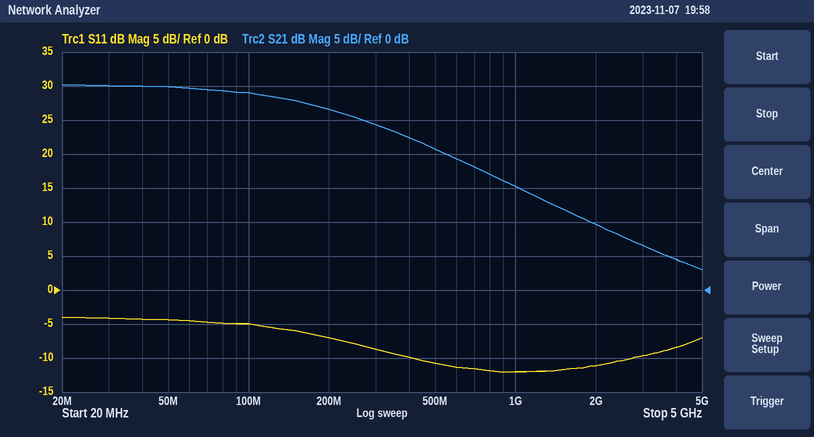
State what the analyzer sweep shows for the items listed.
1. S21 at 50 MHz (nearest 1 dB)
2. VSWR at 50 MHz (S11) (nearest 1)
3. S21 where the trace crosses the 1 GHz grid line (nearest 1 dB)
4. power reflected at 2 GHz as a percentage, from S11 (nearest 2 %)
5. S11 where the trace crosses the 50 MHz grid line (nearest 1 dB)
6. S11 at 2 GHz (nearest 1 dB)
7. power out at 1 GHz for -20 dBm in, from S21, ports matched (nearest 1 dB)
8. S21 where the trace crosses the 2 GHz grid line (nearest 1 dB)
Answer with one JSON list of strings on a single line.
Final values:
["30 dB", "4", "15 dB", "8 %", "-4 dB", "-11 dB", "-5 dBm", "10 dB"]
